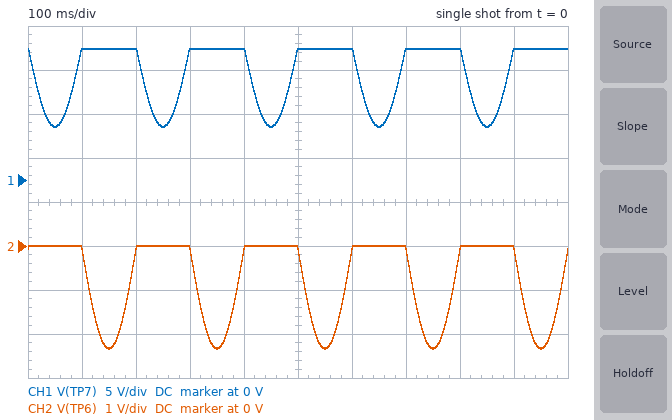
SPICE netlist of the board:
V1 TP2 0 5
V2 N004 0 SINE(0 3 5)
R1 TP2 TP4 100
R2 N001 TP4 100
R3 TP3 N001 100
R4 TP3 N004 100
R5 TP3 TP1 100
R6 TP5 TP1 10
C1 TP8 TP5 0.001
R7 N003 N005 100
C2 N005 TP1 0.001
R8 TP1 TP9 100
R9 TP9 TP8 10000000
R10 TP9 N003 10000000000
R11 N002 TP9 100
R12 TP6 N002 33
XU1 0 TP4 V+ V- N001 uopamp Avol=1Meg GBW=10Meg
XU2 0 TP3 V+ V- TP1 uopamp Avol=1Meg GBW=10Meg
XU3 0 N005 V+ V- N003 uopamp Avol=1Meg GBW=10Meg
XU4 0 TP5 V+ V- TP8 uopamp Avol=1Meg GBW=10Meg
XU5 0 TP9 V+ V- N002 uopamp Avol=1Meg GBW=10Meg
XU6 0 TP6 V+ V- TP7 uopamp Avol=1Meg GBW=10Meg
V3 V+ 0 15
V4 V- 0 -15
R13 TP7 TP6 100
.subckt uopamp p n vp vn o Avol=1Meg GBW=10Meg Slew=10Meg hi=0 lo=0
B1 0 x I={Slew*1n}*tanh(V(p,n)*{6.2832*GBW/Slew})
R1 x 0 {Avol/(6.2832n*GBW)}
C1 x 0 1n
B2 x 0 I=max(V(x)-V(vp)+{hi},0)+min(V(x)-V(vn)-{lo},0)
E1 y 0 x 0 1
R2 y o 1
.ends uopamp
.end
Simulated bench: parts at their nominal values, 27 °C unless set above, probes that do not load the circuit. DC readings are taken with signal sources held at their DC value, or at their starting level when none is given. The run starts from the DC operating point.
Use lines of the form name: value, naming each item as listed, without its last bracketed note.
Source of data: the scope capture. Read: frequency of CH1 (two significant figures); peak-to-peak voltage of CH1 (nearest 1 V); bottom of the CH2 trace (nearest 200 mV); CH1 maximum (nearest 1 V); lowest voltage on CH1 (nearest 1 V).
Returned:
frequency of CH1: 5.0 Hz
peak-to-peak voltage of CH1: 9 V
bottom of the CH2 trace: -2.4 V
CH1 maximum: 15 V
lowest voltage on CH1: 6 V
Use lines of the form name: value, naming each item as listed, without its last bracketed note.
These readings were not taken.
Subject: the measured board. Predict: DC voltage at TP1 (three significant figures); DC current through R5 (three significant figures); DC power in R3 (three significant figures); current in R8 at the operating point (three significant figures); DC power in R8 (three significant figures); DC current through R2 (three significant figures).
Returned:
DC voltage at TP1: 5.00 V
DC current through R5: 50.0 mA
DC power in R3: 250 mW
current in R8 at the operating point: 50.0 mA
DC power in R8: 250 mW
DC current through R2: 50.0 mA
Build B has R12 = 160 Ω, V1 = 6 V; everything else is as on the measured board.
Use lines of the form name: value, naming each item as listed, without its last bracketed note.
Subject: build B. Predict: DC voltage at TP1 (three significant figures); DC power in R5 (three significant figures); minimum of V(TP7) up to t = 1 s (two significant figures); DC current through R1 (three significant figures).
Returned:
DC voltage at TP1: 6.00 V
DC power in R5: 360 mW
minimum of V(TP7) up to t = 1 s: 1.9 V
DC current through R1: 60.0 mA
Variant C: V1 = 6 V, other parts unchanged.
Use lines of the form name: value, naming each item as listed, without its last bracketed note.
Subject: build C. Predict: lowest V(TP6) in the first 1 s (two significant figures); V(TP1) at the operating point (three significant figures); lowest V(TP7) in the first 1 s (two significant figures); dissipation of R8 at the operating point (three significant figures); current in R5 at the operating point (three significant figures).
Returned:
lowest V(TP6) in the first 1 s: -3.1 V
V(TP1) at the operating point: 6.00 V
lowest V(TP7) in the first 1 s: 9.1 V
dissipation of R8 at the operating point: 360 mW
current in R5 at the operating point: 60.0 mA
